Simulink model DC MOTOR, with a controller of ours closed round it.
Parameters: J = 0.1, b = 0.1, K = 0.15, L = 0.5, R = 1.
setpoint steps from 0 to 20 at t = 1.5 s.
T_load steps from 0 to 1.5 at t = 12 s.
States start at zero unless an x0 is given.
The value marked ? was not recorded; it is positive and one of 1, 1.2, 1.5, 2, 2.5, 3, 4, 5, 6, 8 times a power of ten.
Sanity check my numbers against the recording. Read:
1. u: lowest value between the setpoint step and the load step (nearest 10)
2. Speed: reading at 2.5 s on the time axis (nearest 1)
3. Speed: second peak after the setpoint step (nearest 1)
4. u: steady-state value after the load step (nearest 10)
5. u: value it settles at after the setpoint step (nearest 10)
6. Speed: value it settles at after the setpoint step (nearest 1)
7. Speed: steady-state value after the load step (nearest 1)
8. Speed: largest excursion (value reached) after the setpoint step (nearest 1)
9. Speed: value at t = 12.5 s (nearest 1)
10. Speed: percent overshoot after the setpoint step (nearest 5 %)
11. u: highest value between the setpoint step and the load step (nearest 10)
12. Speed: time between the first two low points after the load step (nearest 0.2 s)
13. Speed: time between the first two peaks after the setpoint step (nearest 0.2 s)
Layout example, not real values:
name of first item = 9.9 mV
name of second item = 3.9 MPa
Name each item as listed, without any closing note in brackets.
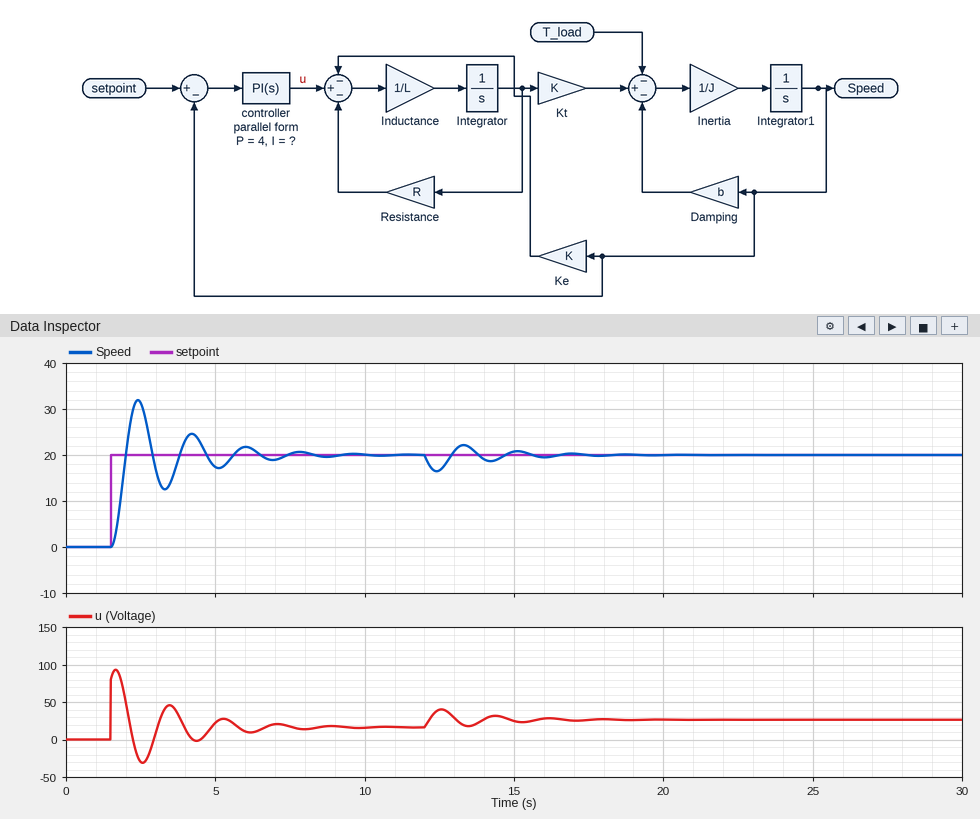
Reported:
u: lowest value between the setpoint step and the load step = -30
Speed: reading at 2.5 s on the time axis = 31
Speed: second peak after the setpoint step = 25
u: steady-state value after the load step = 30
u: value it settles at after the setpoint step = 20
Speed: value it settles at after the setpoint step = 20
Speed: steady-state value after the load step = 20
Speed: largest excursion (value reached) after the setpoint step = 32
Speed: value at t = 12.5 s = 17
Speed: percent overshoot after the setpoint step = 60 %
u: highest value between the setpoint step and the load step = 90
Speed: time between the first two low points after the load step = 1.8 s
Speed: time between the first two peaks after the setpoint step = 1.8 s
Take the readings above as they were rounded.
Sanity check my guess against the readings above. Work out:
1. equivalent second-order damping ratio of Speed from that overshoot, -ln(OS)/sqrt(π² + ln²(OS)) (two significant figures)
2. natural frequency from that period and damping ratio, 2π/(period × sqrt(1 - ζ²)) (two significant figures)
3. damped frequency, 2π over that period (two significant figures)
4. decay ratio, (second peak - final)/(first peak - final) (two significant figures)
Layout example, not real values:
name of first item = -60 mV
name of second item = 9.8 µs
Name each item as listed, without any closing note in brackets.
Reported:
equivalent second-order damping ratio of Speed from that overshoot, -ln(OS)/sqrt(π² + ln²(OS)) = 0.16
natural frequency from that period and damping ratio, 2π/(period × sqrt(1 - ζ²)) = 3.5 rad/s
damped frequency, 2π over that period = 3.5 rad/s
decay ratio, (second peak - final)/(first peak - final) = 0.42
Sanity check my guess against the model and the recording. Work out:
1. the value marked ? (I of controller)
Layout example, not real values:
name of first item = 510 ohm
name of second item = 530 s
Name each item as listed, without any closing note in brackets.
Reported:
the value marked ? = 8
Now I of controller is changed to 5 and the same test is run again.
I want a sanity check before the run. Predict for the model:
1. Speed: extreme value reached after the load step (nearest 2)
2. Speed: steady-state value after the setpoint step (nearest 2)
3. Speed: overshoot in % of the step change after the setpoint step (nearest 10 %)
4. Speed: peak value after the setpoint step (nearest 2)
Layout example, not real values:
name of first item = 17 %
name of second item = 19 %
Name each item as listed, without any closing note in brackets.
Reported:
Speed: extreme value reached after the load step = 16
Speed: steady-state value after the setpoint step = 20
Speed: overshoot in % of the step change after the setpoint step = 40 %
Speed: peak value after the setpoint step = 28
